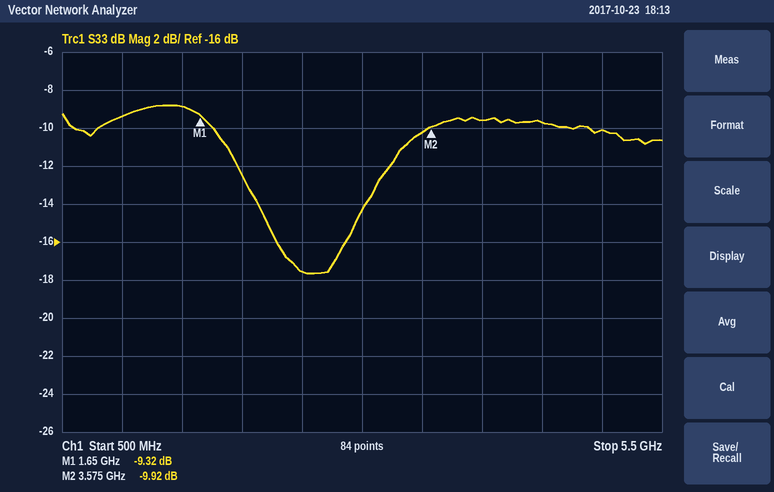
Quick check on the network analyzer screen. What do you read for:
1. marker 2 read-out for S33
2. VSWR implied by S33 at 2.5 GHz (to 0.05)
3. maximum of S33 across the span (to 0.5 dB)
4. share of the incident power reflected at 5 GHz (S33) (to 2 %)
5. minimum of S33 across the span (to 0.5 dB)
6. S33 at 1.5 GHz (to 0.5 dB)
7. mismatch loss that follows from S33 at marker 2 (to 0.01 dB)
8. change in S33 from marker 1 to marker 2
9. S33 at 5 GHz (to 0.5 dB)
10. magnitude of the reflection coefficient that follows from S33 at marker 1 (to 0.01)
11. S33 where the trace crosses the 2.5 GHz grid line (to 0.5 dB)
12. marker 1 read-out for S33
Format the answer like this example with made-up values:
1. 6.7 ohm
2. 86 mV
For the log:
1. -9.92 dB
2. 1.30
3. -9.0 dB
4. 10 %
5. -17.5 dB
6. -9.0 dB
7. 0.47 dB
8. -0.60 dB
9. -10.0 dB
10. 0.34
11. -17.5 dB
12. -9.32 dB
